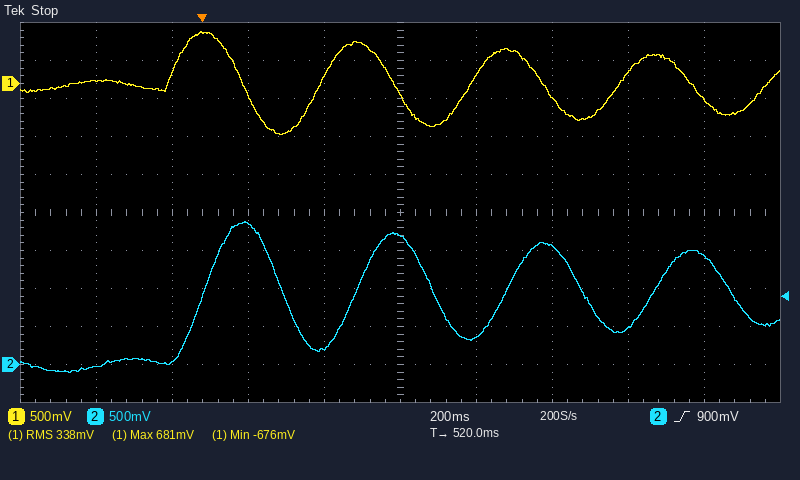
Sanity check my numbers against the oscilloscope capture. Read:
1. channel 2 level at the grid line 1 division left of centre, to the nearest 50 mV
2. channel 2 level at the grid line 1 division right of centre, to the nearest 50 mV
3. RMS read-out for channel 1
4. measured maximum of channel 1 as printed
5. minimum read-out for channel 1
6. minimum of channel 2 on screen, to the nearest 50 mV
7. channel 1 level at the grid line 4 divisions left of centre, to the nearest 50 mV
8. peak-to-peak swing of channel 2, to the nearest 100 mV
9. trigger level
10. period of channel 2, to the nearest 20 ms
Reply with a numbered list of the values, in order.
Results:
1. 200 mV
2. 350 mV
3. 338 mV
4. 681 mV
5. -676 mV
6. -100 mV
7. 50 mV
8. 2.00 V
9. 900 mV
10. 400 ms
